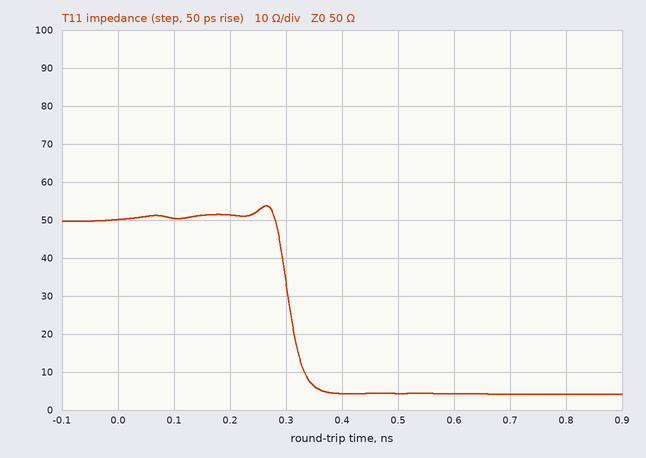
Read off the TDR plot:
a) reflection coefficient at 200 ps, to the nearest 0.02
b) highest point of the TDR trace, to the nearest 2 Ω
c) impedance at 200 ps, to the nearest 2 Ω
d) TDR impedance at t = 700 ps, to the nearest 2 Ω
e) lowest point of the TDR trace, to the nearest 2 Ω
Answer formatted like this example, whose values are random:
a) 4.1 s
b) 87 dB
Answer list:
a) +0.02
b) 54 Ω
c) 52 Ω
d) 4 Ω
e) 4 Ω
